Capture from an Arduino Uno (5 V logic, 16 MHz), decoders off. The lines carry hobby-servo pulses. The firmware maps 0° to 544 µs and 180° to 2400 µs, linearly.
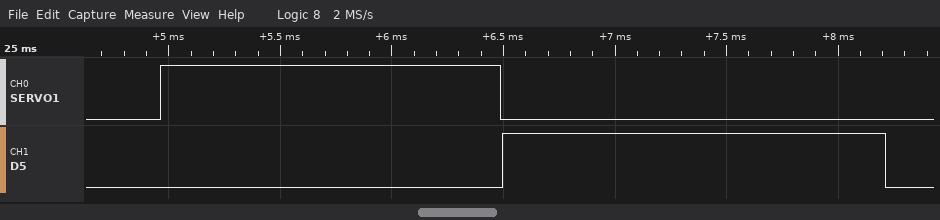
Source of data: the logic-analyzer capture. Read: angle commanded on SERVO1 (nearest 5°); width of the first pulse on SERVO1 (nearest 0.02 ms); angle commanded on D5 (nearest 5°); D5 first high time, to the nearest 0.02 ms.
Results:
95°
1.52 ms
115°
1.72 ms
